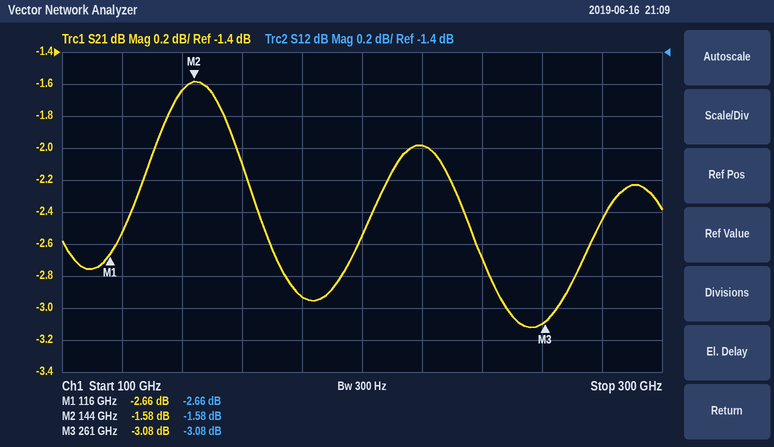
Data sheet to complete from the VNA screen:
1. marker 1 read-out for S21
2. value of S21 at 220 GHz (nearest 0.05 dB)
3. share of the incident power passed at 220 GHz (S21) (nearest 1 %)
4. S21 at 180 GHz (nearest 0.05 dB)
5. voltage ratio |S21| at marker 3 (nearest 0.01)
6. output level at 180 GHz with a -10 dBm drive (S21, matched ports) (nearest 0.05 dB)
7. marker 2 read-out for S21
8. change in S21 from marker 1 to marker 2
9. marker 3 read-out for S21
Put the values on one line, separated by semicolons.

-2.66 dB; -2.00 dB; 63 %; -2.95 dB; 0.70; -12.95 dBm; -1.58 dB; 1.08 dB; -3.08 dB
